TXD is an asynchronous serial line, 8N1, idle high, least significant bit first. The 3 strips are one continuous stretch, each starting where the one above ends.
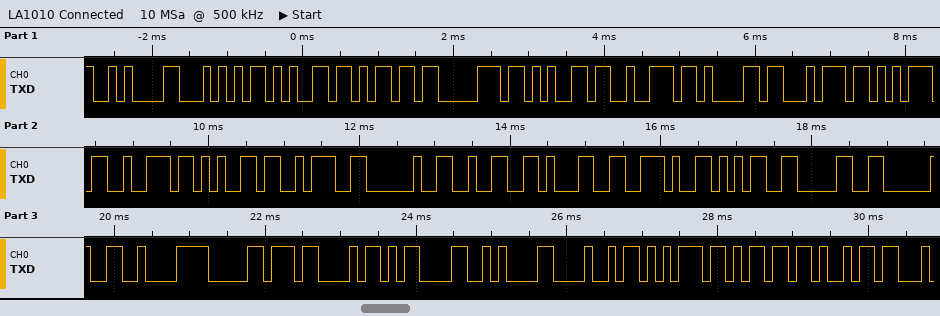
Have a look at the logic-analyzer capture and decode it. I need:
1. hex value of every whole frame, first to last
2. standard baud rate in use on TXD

0x0A 0x54 0x65 0x6D 0x70 0x65 0x72 0x61 0x74 0x75 0x72 0x65 0x3A 0x20 0x32 0x31 0x2E 0x35 0x30 0x20 0xC2 0xB0 0x43 0x0D 0x0A 0x48 0x75 0x6D 0x69
9600 baud
